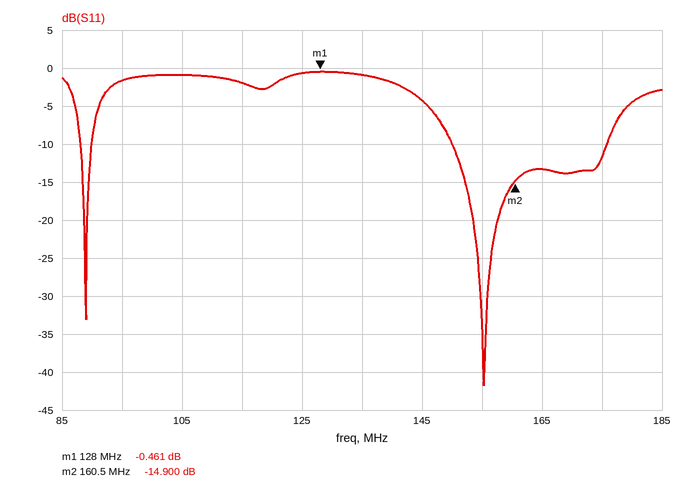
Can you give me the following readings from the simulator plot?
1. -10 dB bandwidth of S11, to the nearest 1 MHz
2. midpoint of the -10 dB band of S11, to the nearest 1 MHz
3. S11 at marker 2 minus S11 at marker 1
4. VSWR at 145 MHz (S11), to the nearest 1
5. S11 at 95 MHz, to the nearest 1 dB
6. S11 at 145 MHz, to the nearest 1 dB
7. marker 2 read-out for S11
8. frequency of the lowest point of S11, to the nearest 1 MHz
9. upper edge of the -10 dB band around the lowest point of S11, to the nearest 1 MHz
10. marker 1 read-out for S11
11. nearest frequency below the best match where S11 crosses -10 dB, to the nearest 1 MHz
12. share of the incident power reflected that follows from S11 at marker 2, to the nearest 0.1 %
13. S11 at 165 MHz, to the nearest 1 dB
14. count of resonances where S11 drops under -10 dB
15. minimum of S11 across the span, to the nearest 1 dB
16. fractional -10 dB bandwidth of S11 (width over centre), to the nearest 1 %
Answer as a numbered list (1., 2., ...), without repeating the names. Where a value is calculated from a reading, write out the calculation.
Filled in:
1. 176 MHz − 150 MHz = 26 MHz
2. 163 MHz
3. -14.9 − (-0.461) = -14.439 dB
4. |Γ| = 10^(-4/20) = 0.6310; VSWR = (1 + 0.6310)/(1 − 0.6310) ≈ 4
5. -2 dB
6. -4 dB
7. -14.900 dB
8. 155 MHz
9. 176 MHz
10. -0.461 dB
11. 150 MHz
12. 10^(-14.9/10) ≈ 3.2 %
13. -13 dB
14. 2
15. -42 dB
16. 26 MHz / 163 MHz ≈ 16 %
